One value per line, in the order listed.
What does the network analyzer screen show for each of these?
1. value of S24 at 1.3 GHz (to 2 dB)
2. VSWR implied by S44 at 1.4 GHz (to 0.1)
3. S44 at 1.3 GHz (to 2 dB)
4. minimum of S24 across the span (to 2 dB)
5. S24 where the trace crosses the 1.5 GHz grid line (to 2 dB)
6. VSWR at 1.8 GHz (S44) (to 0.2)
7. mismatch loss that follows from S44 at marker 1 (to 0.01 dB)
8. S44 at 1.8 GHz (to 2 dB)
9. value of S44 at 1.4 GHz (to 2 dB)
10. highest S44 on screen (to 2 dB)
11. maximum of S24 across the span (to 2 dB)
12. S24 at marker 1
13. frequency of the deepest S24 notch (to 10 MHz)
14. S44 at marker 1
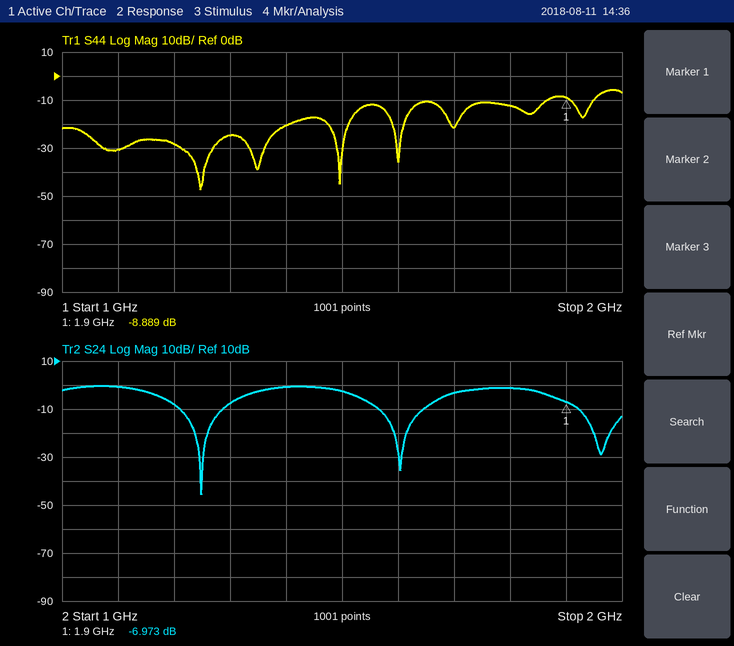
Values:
-8 dB
1.2
-24 dB
-46 dB
-2 dB
1.6
0.60 dB
-12 dB
-20 dB
-6 dB
0 dB
-6.973 dB
1.25 GHz
-8.889 dB
